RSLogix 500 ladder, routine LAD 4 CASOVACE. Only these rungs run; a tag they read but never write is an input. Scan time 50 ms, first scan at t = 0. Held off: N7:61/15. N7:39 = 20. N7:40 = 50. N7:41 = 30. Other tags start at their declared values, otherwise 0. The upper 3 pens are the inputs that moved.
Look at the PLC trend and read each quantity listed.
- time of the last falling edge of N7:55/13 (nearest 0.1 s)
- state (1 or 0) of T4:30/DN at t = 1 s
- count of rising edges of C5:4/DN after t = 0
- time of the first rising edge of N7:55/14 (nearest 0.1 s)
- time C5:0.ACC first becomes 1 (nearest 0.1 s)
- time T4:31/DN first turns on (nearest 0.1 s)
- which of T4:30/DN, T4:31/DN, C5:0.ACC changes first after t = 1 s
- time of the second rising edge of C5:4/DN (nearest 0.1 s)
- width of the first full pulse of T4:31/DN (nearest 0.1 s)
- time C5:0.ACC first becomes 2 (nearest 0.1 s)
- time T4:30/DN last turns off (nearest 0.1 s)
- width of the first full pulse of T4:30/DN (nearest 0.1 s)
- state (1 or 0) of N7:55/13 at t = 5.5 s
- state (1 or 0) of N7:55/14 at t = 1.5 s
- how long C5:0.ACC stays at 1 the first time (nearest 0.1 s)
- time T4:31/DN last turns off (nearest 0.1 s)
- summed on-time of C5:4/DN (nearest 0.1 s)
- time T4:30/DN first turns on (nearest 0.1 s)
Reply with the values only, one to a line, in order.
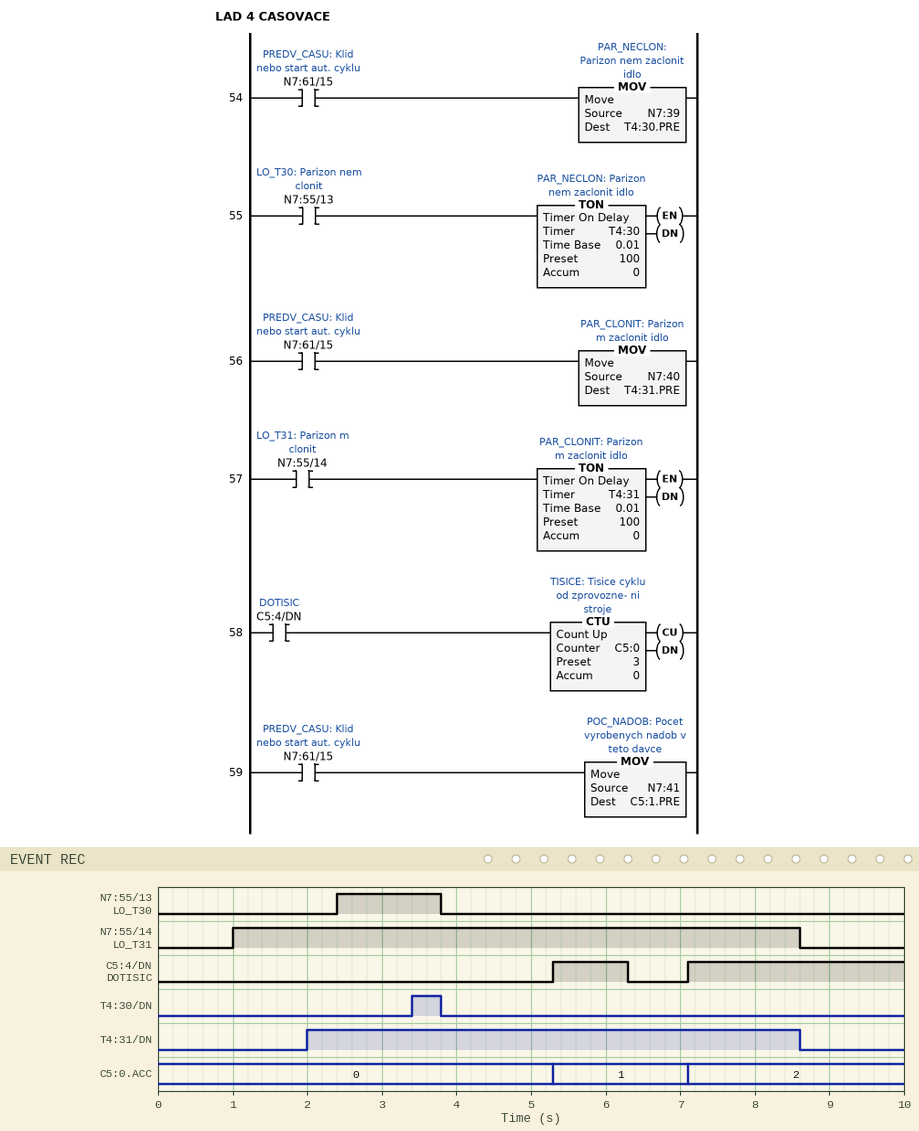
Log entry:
3.8 s
0
2
1.0 s
5.3 s
2.0 s
T4:31/DN
7.1 s
6.6 s
7.1 s
3.8 s
0.4 s
0
1
1.8 s
8.6 s
3.9 s
3.4 s
